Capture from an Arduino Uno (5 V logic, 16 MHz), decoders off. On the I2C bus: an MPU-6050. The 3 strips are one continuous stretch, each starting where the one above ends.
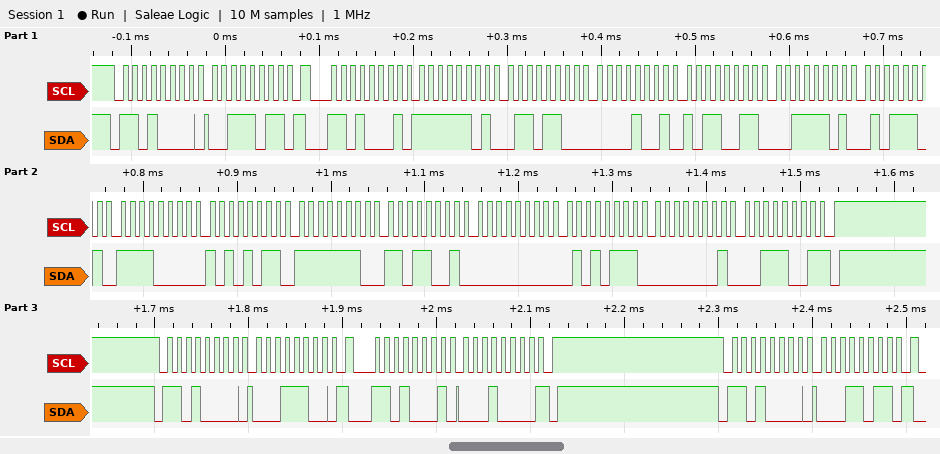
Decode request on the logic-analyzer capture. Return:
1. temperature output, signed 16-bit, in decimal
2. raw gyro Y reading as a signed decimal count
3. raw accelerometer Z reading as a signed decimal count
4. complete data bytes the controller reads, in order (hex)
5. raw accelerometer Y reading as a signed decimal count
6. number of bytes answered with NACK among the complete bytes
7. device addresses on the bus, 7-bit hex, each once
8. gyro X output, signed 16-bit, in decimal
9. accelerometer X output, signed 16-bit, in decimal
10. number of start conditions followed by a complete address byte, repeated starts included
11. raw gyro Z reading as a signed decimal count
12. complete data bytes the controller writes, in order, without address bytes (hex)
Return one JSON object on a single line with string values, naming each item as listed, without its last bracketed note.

{"temperature output, signed 16-bit, in decimal": "-3925", "raw gyro Y reading as a signed decimal count": "87", "raw accelerometer Z reading as a signed decimal count": "15709", "complete data bytes the controller reads, in order": "FD 6C 09 B3 3D 5D F0 AB FE D9 00 57 01 39 10", "raw accelerometer Y reading as a signed decimal count": "2483", "number of bytes answered with NACK among the complete bytes": "2", "device addresses on the bus, 7-bit hex, each once": "0x68", "gyro X output, signed 16-bit, in decimal": "-295", "accelerometer X output, signed 16-bit, in decimal": "-660", "number of start conditions followed by a complete address byte, repeated starts included": "5", "raw gyro Z reading as a signed decimal count": "313", "complete data bytes the controller writes, in order, without address bytes": "3B 1C 1B"}
